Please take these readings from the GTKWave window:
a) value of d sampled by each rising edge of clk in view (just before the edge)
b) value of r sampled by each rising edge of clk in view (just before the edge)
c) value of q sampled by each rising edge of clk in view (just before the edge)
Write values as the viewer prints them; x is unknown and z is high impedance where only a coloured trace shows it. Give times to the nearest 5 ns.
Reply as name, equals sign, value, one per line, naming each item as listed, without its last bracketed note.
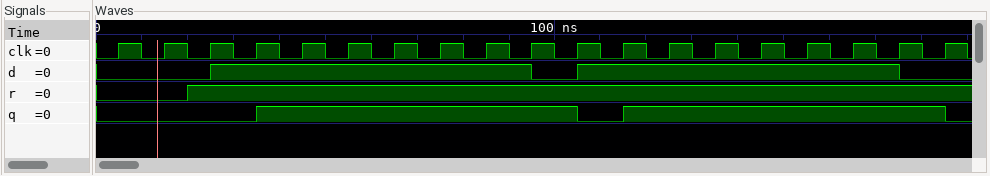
value of d sampled by each rising edge of clk in view = 0 0 0 1 1 1 1 1 1 1 0 1 1 1 1 1 1 1 0
value of r sampled by each rising edge of clk in view = 0 0 1 1 1 1 1 1 1 1 1 1 1 1 1 1 1 1 1
value of q sampled by each rising edge of clk in view = 0 0 0 0 1 1 1 1 1 1 1 0 1 1 1 1 1 1 1
